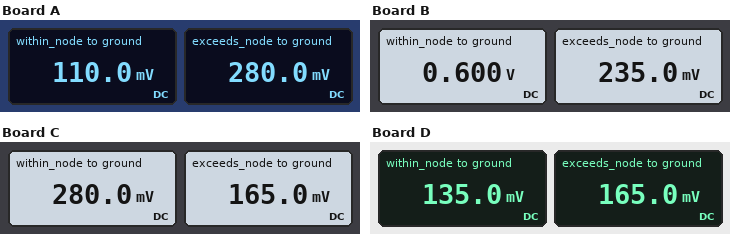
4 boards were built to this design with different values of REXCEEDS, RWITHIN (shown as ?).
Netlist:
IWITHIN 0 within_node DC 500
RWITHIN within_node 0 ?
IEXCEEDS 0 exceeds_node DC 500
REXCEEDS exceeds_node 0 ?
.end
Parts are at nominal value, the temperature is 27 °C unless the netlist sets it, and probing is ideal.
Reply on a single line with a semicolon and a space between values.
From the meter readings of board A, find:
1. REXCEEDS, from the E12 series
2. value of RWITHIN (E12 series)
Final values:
560 µΩ; 220 µΩ
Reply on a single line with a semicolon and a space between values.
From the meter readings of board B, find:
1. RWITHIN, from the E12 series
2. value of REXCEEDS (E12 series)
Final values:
1.2 mΩ; 470 µΩ
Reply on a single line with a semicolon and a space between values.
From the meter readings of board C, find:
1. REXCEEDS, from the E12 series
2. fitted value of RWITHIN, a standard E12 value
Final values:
330 µΩ; 560 µΩ
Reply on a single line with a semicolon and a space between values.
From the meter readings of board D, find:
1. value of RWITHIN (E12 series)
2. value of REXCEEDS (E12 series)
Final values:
270 µΩ; 330 µΩ
